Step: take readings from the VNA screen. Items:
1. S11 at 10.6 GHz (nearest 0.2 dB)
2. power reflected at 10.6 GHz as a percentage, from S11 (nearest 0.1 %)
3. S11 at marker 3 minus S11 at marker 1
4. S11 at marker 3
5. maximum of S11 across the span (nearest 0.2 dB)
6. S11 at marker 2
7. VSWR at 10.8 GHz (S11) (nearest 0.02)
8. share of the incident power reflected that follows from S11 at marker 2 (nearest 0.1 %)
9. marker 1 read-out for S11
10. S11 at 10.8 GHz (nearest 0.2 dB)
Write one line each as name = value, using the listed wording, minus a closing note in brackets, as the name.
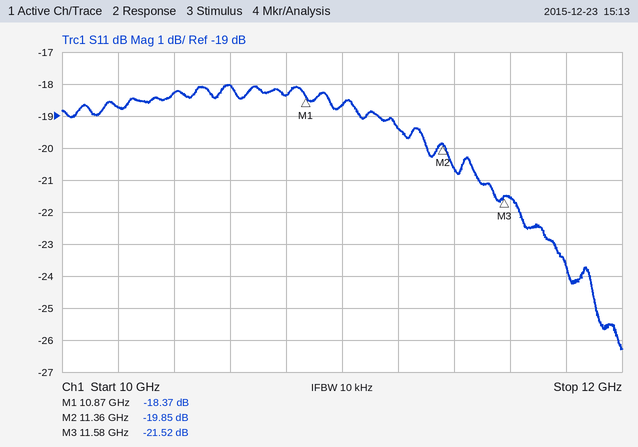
S11 at 10.6 GHz = -18.0 dB
power reflected at 10.6 GHz as a percentage, from S11 = 1.6 %
S11 at marker 3 minus S11 at marker 1 = -3.15 dB
S11 at marker 3 = -21.52 dB
maximum of S11 across the span = -18.0 dB
S11 at marker 2 = -19.85 dB
VSWR at 10.8 GHz (S11) = 1.28
share of the incident power reflected that follows from S11 at marker 2 = 1.0 %
marker 1 read-out for S11 = -18.37 dB
S11 at 10.8 GHz = -18.4 dB
